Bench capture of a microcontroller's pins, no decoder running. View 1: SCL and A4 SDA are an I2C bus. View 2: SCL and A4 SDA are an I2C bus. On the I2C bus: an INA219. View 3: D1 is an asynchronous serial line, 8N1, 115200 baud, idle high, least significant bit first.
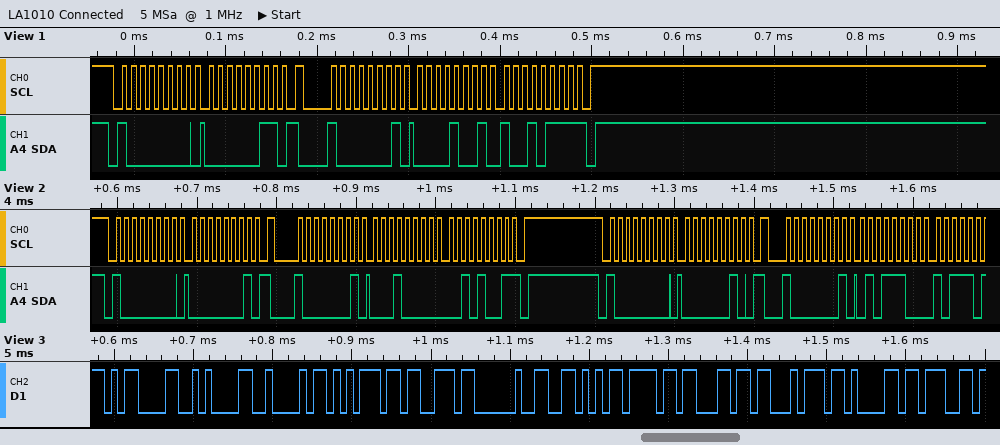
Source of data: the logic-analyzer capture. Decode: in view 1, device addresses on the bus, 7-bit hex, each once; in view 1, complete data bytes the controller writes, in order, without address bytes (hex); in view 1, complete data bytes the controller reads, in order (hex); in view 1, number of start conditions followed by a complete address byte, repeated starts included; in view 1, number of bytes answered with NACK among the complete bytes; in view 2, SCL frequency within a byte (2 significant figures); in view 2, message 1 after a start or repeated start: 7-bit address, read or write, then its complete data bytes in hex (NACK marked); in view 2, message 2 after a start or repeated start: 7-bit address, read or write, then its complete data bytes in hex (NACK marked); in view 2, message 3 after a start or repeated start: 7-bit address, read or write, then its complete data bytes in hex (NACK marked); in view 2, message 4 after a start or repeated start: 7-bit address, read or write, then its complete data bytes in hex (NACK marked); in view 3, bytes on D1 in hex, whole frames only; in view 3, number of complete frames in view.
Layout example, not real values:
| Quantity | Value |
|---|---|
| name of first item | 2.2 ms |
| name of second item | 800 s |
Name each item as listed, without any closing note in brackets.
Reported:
| Quantity | Value |
|---|---|
| in view 1, device addresses on the bus, 7-bit hex, each once | 0x40 |
| in view 1, complete data bytes the controller writes, in order, without address bytes | 03 |
| in view 1, complete data bytes the controller reads, in order | 09 97 |
| in view 1, number of start conditions followed by a complete address byte, repeated starts included | 2 |
| in view 1, number of bytes answered with NACK among the complete bytes | 1 |
| in view 2, SCL frequency within a byte | 100 kHz |
| in view 2, message 1 after a start or repeated start: 7-bit address, read or write, then its complete data bytes in hex | 0x40 write: 01 |
| in view 2, message 2 after a start or repeated start: 7-bit address, read or write, then its complete data bytes in hex | 0x40 read: 10 29 NACK |
| in view 2, message 3 after a start or repeated start: 7-bit address, read or write, then its complete data bytes in hex | 0x40 write: 02 |
| in view 2, message 4 after a start or repeated start: 7-bit address, read or write, then its complete data bytes in hex | 0x40 read: 5C |
| in view 3, bytes on D1 in hex, whole frames only | 0x0D 0x0A 0x42 0x75 0x73 0x20 0x56 0x6F 0x6C 0x74 0x61 0x67 |
| in view 3, number of complete frames in view | 12 |
